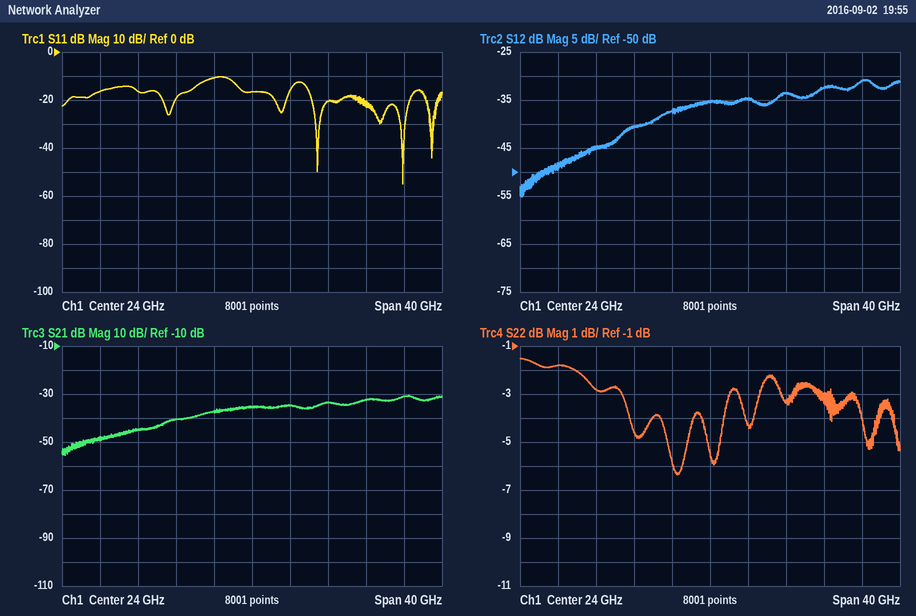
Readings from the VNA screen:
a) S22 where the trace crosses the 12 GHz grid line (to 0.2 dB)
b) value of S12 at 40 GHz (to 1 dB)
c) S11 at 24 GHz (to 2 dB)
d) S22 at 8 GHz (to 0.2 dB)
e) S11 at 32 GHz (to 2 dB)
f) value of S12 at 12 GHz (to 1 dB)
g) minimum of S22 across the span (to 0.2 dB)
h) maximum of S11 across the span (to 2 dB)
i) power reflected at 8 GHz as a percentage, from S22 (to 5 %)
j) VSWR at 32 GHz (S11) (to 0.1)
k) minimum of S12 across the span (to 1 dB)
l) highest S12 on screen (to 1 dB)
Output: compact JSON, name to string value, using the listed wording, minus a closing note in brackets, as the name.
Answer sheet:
{"S22 where the trace crosses the 12 GHz grid line": "-2.8 dB", "value of S12 at 40 GHz": "-31 dB", "S11 at 24 GHz": "-16 dB", "S22 at 8 GHz": "-1.8 dB", "S11 at 32 GHz": "-20 dB", "value of S12 at 12 GHz": "-45 dB", "minimum of S22 across the span": "-6.4 dB", "maximum of S11 across the span": "-10 dB", "power reflected at 8 GHz as a percentage, from S22": "65 %", "VSWR at 32 GHz (S11)": "1.2", "minimum of S12 across the span": "-55 dB", "highest S12 on screen": "-31 dB"}
